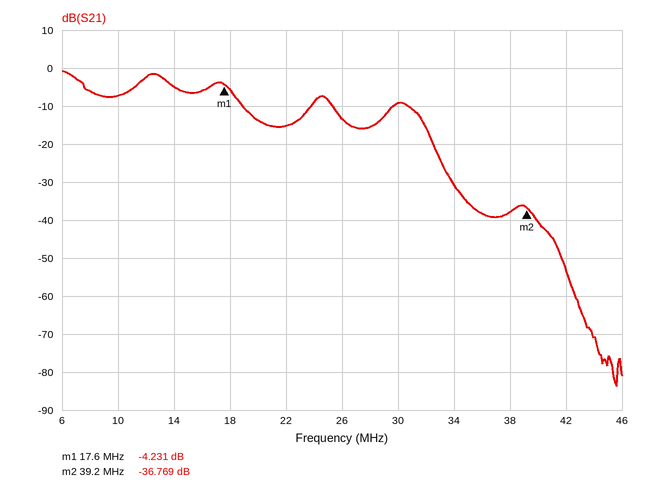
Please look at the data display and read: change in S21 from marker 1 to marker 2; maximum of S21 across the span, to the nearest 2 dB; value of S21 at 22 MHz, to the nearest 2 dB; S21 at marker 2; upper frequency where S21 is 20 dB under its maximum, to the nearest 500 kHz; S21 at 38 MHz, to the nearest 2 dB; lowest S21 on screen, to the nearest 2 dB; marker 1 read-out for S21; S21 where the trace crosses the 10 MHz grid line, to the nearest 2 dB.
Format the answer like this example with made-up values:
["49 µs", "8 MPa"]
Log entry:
["-32.538 dB", "0 dB", "-16 dB", "-36.769 dB", "32.5 MHz", "-38 dB", "-84 dB", "-4.231 dB", "-8 dB"]
